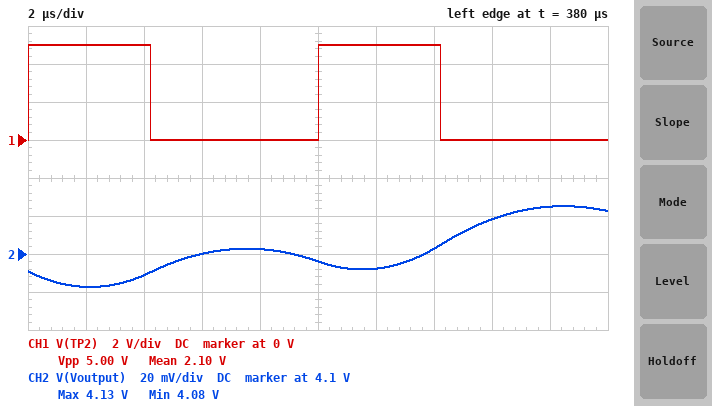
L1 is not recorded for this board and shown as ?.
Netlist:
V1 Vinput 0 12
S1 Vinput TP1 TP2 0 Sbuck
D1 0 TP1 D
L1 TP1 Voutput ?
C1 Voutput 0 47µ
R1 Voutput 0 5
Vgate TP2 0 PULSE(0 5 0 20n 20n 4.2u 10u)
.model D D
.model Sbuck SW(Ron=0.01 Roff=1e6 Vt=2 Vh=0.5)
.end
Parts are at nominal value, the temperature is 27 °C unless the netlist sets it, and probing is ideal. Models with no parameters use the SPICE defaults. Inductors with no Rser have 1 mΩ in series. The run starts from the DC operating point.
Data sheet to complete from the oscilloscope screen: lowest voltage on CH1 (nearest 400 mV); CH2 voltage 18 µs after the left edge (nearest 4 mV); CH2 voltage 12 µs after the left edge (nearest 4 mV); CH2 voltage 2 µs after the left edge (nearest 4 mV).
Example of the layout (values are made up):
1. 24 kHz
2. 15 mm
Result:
1. 0 V
2. 4.124 V
3. 4.092 V
4. 4.084 V
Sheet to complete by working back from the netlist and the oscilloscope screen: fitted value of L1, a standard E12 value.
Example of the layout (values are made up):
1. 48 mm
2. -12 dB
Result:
1. 47 µH
